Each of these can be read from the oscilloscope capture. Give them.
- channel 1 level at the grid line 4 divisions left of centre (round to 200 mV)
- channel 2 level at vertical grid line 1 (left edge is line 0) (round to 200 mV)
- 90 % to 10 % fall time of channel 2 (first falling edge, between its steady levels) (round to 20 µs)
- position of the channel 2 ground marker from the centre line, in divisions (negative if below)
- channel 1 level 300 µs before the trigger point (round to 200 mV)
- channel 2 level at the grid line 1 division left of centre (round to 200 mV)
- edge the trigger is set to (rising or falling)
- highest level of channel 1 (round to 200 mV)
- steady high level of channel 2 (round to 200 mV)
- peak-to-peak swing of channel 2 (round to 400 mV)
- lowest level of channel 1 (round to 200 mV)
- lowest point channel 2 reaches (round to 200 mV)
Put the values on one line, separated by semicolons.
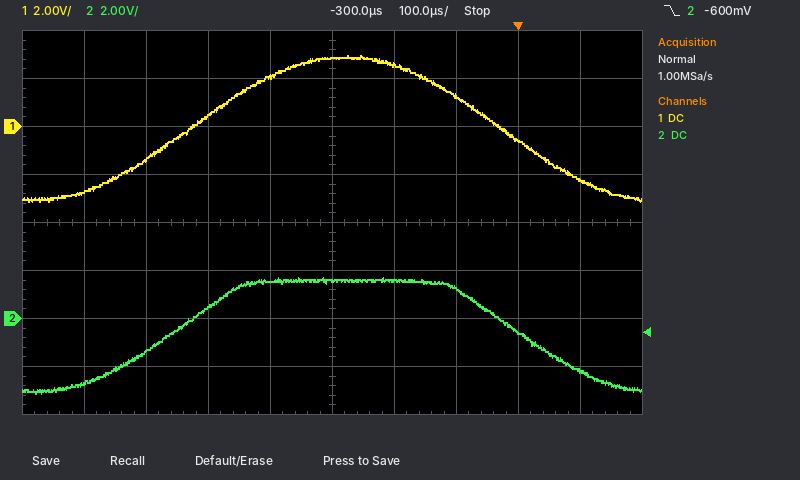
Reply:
-2.8 V; -2.6 V; 220 µs; -2.0 div; 2.8 V; 1.6 V; falling; 3.0 V; 1.6 V; 4.8 V; -3.2 V; -3.2 V
